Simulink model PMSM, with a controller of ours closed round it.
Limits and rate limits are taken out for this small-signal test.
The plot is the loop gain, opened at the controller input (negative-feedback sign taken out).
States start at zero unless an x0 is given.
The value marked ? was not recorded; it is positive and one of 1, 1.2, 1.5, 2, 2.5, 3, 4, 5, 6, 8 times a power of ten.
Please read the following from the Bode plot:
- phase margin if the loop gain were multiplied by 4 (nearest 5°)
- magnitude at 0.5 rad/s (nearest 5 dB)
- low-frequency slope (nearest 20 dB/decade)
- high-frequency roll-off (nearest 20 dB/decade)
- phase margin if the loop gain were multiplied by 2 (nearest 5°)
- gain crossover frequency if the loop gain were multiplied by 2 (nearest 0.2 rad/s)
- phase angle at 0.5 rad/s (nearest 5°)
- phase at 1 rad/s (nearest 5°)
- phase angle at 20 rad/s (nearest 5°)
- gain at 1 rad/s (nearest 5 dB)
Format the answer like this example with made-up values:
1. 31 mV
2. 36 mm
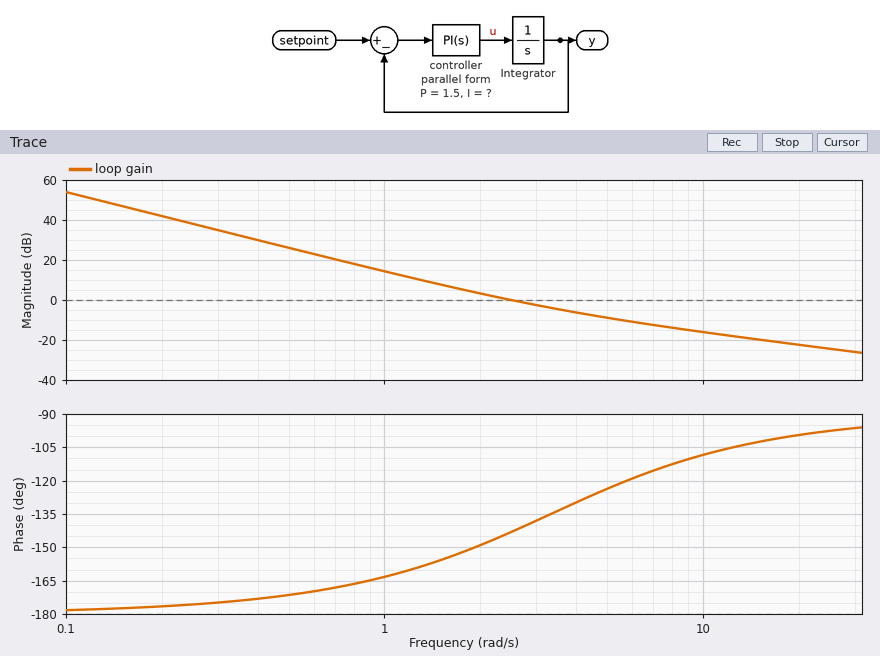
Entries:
1. 65°
2. 25 dB
3. -40 dB/decade
4. -20 dB/decade
5. 50°
6. 4.0 rad/s
7. -170°
8. -165°
9. -100°
10. 15 dB
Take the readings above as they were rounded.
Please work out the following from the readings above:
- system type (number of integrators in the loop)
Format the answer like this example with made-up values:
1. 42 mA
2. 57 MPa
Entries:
1. 2
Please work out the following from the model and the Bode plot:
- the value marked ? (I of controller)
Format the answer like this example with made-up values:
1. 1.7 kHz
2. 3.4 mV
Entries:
1. 5
